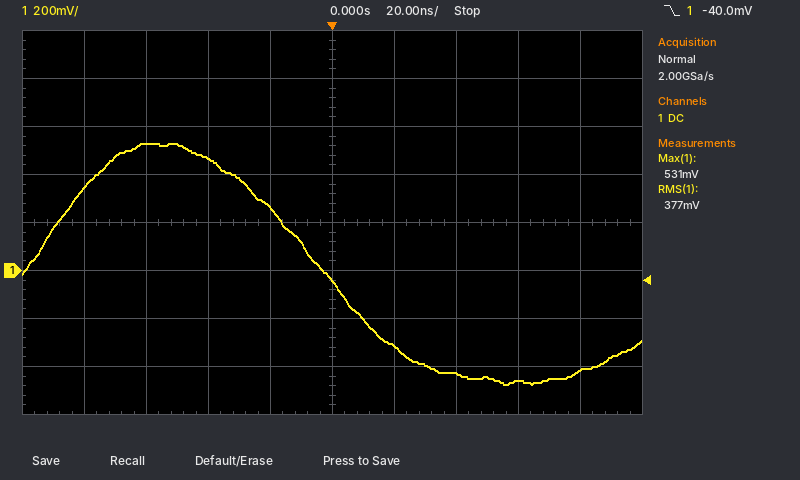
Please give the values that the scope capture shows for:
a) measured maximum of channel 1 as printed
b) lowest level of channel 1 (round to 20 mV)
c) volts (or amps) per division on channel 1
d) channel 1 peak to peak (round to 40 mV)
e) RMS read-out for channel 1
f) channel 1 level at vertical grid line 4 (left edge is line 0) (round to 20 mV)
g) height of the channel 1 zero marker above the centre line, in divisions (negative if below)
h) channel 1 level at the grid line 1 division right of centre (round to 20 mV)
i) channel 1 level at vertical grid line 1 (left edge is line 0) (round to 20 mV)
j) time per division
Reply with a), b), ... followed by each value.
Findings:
a) 531 mV
b) -480 mV
c) 200 mV
d) 1.00 V
e) 377 mV
f) 260 mV
g) -1.0 div
h) -320 mV
i) 340 mV
j) 20 ns
